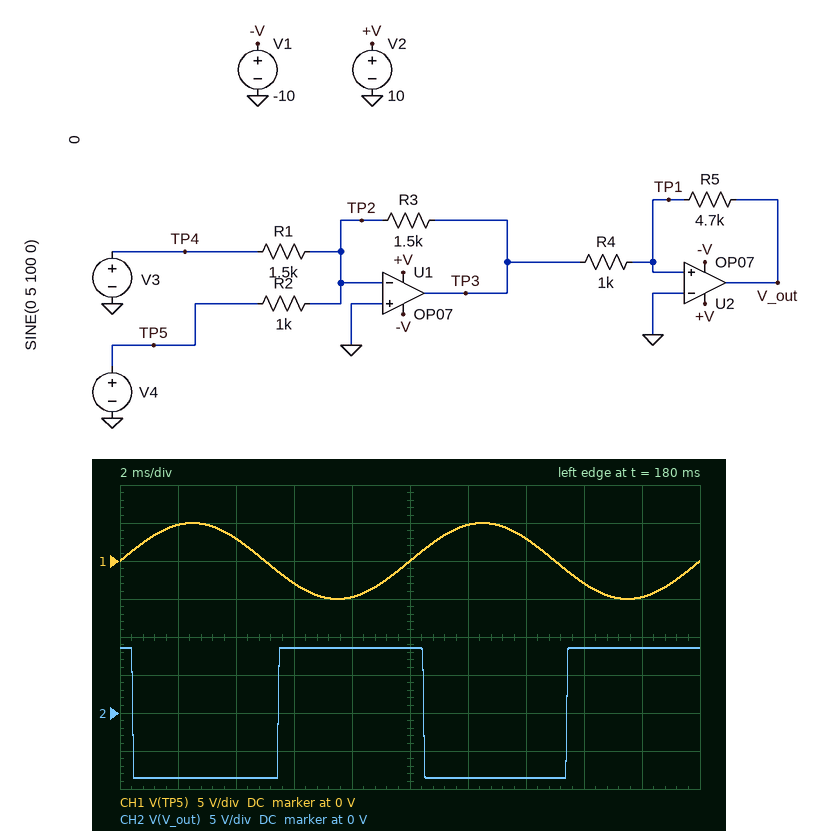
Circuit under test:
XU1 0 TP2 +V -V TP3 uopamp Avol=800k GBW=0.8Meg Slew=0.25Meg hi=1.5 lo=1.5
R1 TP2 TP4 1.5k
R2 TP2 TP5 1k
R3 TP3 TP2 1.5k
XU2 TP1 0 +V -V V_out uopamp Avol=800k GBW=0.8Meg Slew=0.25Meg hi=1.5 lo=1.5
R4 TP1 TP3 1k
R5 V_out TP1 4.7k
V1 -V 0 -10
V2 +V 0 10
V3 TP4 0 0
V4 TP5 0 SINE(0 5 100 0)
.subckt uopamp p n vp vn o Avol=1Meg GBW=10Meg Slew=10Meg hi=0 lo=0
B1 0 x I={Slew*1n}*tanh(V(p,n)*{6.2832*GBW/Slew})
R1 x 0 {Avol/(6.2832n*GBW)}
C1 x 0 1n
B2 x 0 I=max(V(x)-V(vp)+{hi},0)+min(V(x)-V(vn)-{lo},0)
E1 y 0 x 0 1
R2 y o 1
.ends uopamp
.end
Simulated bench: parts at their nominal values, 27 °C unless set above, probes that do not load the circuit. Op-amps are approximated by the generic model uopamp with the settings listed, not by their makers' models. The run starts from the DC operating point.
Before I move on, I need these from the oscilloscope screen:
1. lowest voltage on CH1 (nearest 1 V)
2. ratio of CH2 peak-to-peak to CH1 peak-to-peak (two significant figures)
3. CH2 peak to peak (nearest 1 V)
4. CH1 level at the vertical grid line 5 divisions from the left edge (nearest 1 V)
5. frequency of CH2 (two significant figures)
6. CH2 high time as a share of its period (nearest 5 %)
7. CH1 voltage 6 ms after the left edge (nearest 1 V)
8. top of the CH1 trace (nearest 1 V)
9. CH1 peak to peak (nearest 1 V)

-5 V
1.7
17 V
0 V
100 Hz
50 %
-3 V
5 V
10 V
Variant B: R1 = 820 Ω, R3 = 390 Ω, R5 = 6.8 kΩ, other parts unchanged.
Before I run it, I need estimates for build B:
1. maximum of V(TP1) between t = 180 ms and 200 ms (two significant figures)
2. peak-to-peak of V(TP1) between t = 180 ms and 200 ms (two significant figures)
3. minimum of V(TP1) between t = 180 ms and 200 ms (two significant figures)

2.8 V
5.6 V
-2.8 V
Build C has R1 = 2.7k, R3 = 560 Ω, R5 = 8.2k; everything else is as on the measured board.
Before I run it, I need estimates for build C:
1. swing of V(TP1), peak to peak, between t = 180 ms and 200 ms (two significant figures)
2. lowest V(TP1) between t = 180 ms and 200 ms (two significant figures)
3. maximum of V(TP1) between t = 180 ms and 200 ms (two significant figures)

6.8 V
-3.4 V
3.4 V
